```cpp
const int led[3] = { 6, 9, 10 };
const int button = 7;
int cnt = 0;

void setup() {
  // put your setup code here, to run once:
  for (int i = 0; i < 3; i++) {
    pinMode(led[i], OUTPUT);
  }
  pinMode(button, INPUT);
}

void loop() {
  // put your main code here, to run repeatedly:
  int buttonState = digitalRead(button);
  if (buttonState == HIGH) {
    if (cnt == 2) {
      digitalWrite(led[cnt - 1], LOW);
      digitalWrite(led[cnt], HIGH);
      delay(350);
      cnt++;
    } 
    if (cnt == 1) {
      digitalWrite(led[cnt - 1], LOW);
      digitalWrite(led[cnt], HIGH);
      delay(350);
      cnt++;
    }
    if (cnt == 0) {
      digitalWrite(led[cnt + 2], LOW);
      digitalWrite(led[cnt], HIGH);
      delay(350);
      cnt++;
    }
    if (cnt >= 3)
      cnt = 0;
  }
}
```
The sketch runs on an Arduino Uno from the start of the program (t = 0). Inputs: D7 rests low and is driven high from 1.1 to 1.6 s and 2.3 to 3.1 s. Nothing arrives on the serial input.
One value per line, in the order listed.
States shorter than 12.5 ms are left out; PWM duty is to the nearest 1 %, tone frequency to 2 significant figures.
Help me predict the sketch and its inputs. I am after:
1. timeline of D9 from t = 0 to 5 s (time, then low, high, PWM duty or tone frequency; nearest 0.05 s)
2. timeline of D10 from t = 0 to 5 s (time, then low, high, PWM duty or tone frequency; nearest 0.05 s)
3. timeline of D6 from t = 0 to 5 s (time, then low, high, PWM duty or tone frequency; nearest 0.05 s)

0 s low; 1.45 s high; 2.3 s low; 3 s high
0 s low; 2.3 s high; 2.65 s low
0 s low; 1.1 s high; 1.45 s low; 2.65 s high; 3 s low
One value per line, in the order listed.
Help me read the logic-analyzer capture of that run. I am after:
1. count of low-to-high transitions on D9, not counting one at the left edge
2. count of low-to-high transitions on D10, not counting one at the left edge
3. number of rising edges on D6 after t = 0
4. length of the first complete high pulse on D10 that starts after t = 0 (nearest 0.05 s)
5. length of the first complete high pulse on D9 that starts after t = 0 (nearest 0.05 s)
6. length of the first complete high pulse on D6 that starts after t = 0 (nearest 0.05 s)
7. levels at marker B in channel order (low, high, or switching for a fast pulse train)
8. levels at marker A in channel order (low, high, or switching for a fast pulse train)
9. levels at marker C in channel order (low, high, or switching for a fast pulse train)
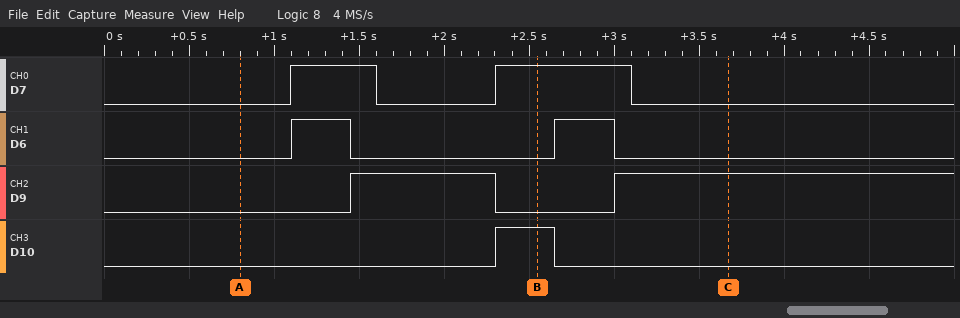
2
1
2
0.35 s
0.85 s
0.35 s
D7 high, D6 low, D9 low, D10 high
D7 low, D6 low, D9 low, D10 low
D7 low, D6 low, D9 high, D10 low
